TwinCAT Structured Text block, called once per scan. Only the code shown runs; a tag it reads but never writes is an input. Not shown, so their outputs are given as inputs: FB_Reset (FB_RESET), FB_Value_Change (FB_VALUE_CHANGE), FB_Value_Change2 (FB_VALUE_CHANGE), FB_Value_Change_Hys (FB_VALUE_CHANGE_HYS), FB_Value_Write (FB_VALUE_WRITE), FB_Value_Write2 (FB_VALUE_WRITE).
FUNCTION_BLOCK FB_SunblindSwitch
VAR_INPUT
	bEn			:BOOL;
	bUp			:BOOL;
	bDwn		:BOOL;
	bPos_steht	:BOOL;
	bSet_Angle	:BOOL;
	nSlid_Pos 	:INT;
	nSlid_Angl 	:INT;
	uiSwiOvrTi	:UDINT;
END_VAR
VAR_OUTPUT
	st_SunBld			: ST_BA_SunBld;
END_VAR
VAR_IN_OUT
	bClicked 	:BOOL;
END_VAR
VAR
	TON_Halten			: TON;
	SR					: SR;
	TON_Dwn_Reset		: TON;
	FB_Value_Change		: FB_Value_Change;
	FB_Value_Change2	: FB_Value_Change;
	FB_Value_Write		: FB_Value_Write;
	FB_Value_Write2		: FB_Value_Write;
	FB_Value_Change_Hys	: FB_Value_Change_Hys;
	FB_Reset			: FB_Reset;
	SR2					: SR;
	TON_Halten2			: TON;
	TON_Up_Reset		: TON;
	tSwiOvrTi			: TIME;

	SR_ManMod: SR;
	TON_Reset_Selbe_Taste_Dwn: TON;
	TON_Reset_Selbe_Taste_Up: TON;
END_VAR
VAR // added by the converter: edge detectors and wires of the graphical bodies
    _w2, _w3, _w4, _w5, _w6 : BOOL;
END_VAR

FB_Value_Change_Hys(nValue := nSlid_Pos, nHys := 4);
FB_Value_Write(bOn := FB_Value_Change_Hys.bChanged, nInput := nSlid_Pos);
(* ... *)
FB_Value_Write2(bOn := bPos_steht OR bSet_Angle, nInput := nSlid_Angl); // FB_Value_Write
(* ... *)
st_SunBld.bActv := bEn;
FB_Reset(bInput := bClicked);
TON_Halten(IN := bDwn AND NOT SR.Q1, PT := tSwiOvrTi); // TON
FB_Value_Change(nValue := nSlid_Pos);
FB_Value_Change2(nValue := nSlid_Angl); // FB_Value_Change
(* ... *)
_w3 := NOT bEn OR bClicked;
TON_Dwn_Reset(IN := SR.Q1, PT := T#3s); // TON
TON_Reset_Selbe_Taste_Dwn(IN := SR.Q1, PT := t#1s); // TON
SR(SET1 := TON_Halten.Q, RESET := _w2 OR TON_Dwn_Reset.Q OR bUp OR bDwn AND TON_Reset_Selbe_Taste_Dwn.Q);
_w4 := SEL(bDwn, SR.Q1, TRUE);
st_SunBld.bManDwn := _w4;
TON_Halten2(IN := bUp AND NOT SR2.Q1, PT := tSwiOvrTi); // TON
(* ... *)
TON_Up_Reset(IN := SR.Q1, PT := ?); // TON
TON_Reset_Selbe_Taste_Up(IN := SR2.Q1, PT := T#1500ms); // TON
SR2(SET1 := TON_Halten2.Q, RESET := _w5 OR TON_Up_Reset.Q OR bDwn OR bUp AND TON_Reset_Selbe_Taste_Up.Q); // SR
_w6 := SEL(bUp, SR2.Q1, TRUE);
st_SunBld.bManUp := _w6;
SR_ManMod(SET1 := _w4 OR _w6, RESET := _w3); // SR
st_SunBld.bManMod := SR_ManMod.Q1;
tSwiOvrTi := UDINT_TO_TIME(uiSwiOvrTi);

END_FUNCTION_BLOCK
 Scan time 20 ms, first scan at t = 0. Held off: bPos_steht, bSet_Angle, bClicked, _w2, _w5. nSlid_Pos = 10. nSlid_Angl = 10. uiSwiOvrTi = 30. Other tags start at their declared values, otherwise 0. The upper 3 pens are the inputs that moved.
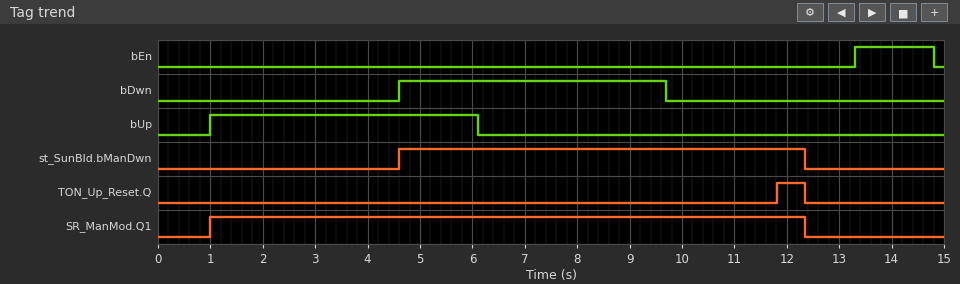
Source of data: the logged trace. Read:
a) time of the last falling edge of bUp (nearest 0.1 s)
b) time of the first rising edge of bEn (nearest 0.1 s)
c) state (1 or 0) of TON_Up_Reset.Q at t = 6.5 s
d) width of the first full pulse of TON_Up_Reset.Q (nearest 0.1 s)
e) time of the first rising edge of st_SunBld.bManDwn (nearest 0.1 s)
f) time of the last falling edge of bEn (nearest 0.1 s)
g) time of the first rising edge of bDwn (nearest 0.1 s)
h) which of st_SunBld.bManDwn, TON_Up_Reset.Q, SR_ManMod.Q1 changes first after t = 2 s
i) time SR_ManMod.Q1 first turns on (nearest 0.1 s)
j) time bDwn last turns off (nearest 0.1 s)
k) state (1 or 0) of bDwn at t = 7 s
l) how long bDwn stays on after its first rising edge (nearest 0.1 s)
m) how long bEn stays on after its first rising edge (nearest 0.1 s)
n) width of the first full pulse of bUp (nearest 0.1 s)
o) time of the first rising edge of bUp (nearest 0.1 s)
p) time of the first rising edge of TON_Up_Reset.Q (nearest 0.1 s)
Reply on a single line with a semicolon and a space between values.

6.1 s; 13.3 s; 0; 0.5 s; 4.6 s; 14.8 s; 4.6 s; st_SunBld.bManDwn; 1.0 s; 9.7 s; 1; 5.1 s; 1.5 s; 5.1 s; 1.0 s; 11.8 s
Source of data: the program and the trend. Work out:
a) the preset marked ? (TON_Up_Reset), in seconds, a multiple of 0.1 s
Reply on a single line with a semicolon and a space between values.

2.5 s
